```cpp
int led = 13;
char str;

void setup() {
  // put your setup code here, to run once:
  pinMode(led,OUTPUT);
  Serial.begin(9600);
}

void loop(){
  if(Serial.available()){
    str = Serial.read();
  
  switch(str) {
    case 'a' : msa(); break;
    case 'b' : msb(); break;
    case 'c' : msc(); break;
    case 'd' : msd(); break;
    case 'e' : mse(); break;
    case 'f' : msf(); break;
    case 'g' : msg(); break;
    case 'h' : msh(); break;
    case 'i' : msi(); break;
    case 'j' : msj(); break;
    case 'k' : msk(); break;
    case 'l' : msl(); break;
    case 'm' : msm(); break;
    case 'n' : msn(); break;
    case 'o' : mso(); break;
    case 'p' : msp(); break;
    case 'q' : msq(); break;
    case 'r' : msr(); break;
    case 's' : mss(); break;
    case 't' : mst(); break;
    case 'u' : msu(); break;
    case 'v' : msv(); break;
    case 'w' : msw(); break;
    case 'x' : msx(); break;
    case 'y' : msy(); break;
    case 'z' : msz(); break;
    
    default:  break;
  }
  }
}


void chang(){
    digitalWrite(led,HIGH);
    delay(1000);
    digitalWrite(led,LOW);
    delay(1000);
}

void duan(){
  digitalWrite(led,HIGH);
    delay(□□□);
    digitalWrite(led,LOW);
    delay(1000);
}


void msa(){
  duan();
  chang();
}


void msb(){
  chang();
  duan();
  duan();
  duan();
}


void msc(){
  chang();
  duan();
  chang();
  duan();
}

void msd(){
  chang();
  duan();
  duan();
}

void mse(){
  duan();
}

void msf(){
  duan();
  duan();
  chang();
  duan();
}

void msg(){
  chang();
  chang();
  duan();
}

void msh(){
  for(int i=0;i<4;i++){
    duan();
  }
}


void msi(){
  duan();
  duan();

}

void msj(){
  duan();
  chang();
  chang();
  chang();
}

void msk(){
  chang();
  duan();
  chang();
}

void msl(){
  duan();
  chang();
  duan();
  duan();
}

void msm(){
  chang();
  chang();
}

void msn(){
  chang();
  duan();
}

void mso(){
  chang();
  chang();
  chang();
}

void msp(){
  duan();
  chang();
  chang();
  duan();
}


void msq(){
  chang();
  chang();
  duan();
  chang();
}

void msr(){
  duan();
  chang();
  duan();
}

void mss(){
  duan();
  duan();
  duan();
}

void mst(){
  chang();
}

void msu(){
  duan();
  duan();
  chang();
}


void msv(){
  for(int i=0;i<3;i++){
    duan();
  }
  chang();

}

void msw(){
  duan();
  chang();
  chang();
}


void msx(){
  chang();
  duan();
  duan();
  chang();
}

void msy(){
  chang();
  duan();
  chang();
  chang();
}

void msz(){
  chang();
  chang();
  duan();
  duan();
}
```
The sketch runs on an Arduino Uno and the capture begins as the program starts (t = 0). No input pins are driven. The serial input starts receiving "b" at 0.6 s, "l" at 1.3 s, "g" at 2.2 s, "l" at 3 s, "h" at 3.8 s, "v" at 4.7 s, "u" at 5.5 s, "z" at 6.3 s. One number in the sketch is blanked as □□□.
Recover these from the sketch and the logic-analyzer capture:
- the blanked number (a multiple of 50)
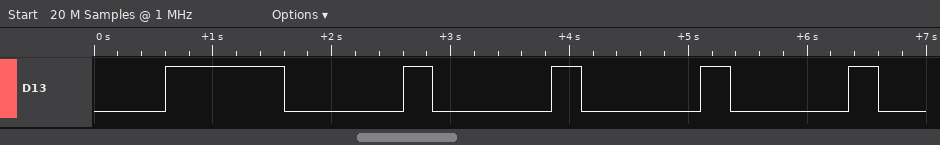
250
